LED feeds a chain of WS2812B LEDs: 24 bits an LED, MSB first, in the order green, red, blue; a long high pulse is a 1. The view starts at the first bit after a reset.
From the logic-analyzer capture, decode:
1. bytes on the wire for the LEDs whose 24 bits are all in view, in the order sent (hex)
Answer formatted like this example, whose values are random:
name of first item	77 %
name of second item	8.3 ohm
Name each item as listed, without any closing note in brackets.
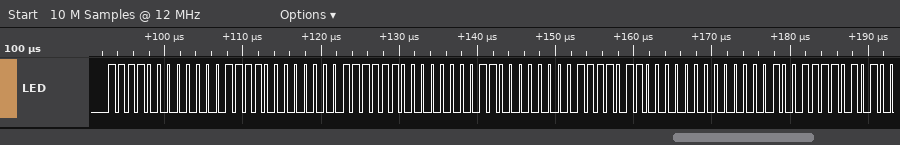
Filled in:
bytes on the wire for the LEDs whose 24 bits are all in view, in the order sent	F0 0F 00 FC 03 00 F6 00 09
